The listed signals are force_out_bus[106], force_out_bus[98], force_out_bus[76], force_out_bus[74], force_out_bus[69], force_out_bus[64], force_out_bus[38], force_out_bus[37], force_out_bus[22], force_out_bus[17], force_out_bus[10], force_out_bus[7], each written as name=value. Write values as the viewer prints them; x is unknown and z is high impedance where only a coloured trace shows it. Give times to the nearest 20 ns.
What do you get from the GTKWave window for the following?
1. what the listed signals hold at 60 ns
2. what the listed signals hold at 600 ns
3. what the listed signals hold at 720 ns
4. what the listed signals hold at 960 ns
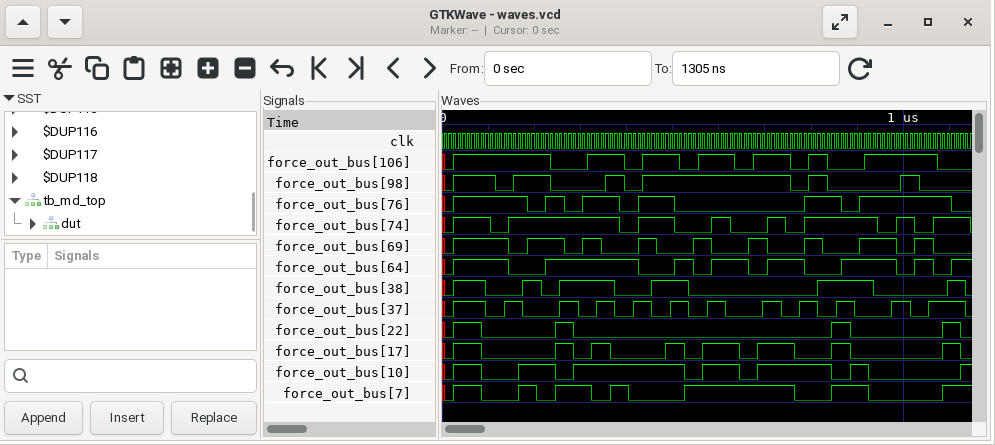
force_out_bus[106]=1, force_out_bus[98]=1, force_out_bus[76]=1, force_out_bus[74]=1, force_out_bus[69]=1, force_out_bus[64]=1, force_out_bus[38]=1, force_out_bus[37]=1, force_out_bus[22]=1, force_out_bus[17]=1, force_out_bus[10]=1, force_out_bus[7]=1
force_out_bus[106]=1, force_out_bus[98]=1, force_out_bus[76]=0, force_out_bus[74]=1, force_out_bus[69]=0, force_out_bus[64]=1, force_out_bus[38]=0, force_out_bus[37]=1, force_out_bus[22]=0, force_out_bus[17]=1, force_out_bus[10]=1, force_out_bus[7]=1
force_out_bus[106]=1, force_out_bus[98]=1, force_out_bus[76]=0, force_out_bus[74]=1, force_out_bus[69]=0, force_out_bus[64]=1, force_out_bus[38]=0, force_out_bus[37]=1, force_out_bus[22]=0, force_out_bus[17]=1, force_out_bus[10]=1, force_out_bus[7]=1
force_out_bus[106]=1, force_out_bus[98]=0, force_out_bus[76]=1, force_out_bus[74]=0, force_out_bus[69]=1, force_out_bus[64]=1, force_out_bus[38]=0, force_out_bus[37]=0, force_out_bus[22]=0, force_out_bus[17]=0, force_out_bus[10]=0, force_out_bus[7]=0
